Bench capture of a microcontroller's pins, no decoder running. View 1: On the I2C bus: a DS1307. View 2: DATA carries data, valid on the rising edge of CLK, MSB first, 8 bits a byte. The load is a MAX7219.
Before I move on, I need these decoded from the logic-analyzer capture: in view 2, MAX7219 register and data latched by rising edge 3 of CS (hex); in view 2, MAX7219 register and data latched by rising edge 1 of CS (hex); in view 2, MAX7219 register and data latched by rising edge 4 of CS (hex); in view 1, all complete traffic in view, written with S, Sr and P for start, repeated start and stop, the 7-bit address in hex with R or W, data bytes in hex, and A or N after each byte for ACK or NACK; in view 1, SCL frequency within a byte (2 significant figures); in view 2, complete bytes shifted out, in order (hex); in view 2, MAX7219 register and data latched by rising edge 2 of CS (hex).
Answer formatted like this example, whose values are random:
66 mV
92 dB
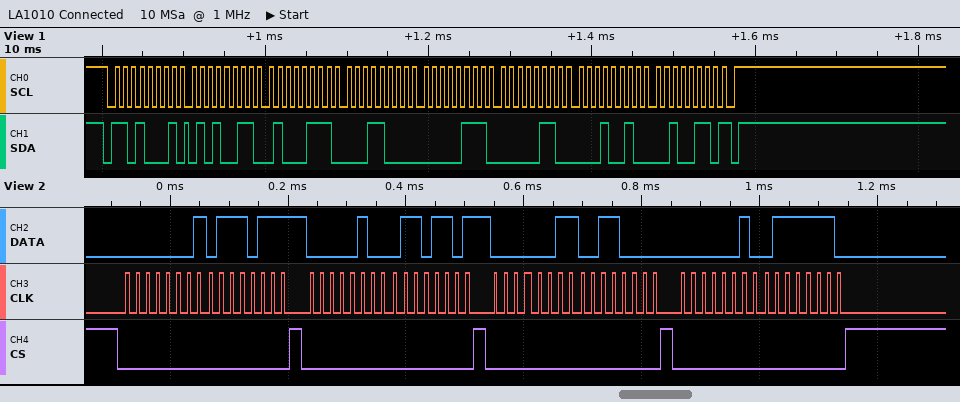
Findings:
register 0x3, data 0x30
register 0x1, data 0x77
register 0x2, data 0x7E
S 68R A 53 A 47 A 18 A 07 A 06 A 12 A 26 N P
100 kHz
0x01 0x77 0x04 0x6D 0x03 0x30 0x02 0x7E
register 0x4, data 0x6D
